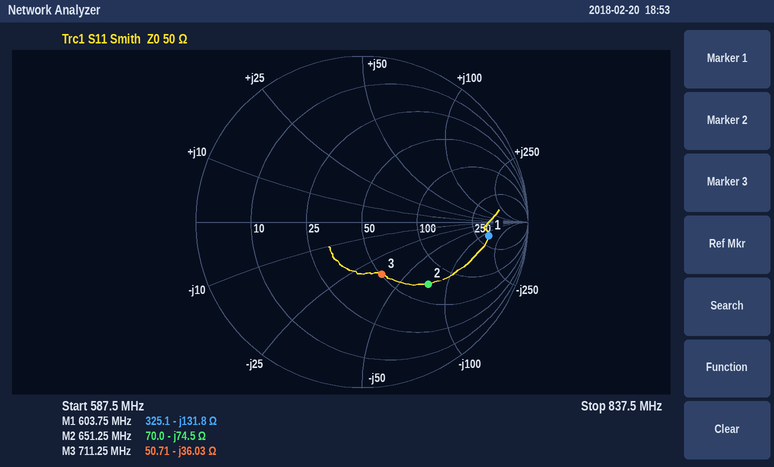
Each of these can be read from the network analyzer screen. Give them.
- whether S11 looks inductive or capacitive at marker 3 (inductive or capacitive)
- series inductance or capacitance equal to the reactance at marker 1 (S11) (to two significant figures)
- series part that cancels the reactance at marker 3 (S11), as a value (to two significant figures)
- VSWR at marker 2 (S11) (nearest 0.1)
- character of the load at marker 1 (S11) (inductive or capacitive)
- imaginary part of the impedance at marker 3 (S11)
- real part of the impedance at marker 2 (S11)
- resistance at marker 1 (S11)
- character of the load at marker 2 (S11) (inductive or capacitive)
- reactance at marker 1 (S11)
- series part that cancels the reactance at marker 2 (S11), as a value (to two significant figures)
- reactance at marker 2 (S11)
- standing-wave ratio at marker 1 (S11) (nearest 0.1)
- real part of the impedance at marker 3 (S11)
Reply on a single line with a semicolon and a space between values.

capacitive; 2.0 pF; 8.1 nH; 3.4; capacitive; -36.03 Ω; 70.0 Ω; 325.1 Ω; capacitive; -131.8 Ω; 18 nH; -74.5 Ω; 7.6; 50.71 Ω
